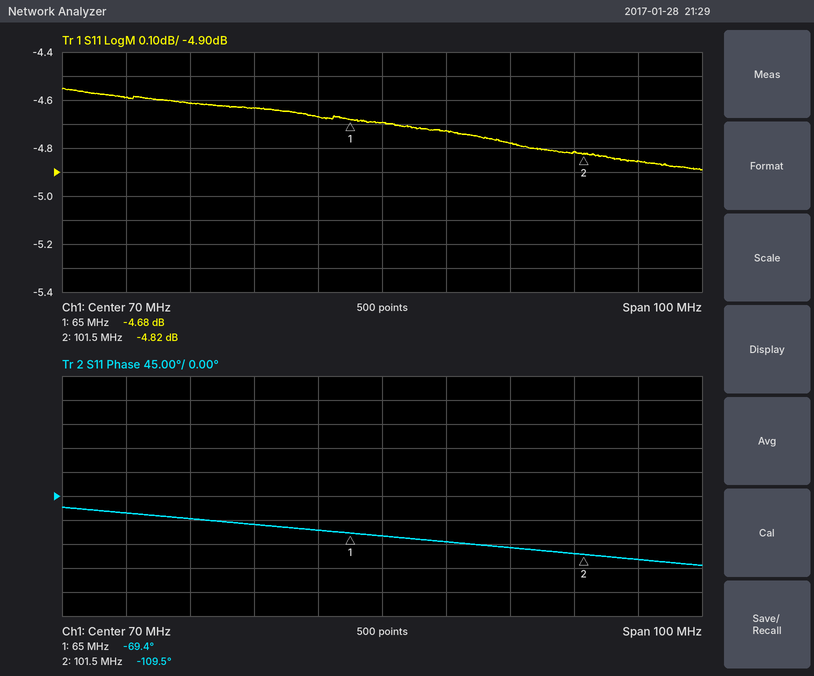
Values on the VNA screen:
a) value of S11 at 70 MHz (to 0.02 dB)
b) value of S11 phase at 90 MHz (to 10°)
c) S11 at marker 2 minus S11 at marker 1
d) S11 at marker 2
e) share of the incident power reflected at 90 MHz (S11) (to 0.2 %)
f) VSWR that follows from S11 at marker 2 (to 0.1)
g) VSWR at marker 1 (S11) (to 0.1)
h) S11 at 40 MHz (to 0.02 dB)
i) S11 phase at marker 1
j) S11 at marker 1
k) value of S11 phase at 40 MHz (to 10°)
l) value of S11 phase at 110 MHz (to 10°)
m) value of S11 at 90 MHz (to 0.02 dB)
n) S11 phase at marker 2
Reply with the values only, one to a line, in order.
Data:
-4.70 dB
-100°
-0.14 dB
-4.82 dB
33.2 %
3.7
3.8
-4.62 dB
-69.4°
-4.68 dB
-40°
-120°
-4.78 dB
-109.5°
